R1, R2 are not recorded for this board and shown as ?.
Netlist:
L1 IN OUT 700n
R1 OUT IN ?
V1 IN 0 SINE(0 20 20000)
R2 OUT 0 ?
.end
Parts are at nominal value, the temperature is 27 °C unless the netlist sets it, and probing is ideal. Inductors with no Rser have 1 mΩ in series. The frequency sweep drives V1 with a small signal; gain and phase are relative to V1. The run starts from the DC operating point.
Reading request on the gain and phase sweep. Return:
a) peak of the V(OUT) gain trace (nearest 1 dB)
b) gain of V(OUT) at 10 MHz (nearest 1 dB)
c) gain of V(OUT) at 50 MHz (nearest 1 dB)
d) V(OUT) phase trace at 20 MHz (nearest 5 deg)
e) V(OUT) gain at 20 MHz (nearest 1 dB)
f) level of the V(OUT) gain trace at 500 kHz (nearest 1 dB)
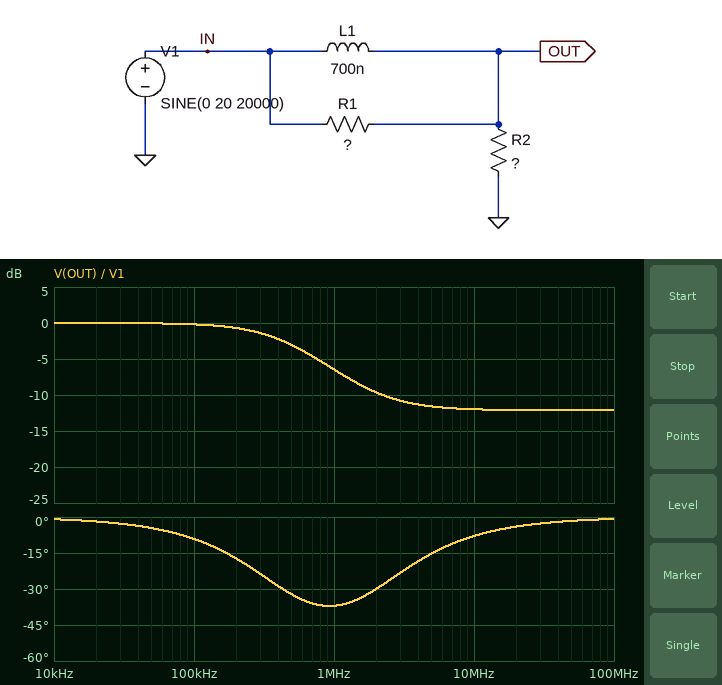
0 dB
-12 dB
-12 dB
-5 deg
-12 dB
-3 dB
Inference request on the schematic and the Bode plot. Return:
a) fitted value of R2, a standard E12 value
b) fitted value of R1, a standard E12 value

2.7 Ω
8.2 Ω
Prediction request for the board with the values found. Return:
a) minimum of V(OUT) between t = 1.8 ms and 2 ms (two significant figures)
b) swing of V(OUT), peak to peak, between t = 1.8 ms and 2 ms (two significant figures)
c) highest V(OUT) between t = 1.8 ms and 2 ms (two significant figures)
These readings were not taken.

-20 V
40 V
20 V
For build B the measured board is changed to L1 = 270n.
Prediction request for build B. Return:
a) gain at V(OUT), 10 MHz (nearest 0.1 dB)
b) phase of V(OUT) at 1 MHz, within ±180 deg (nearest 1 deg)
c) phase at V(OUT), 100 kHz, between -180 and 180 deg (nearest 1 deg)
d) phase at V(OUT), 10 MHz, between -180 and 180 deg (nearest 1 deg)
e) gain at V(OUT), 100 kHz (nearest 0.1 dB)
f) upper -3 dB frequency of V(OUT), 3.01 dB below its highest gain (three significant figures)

-11.3 dB
-28 deg
-4 deg
-19 deg
0 dB
1.28 MHz
